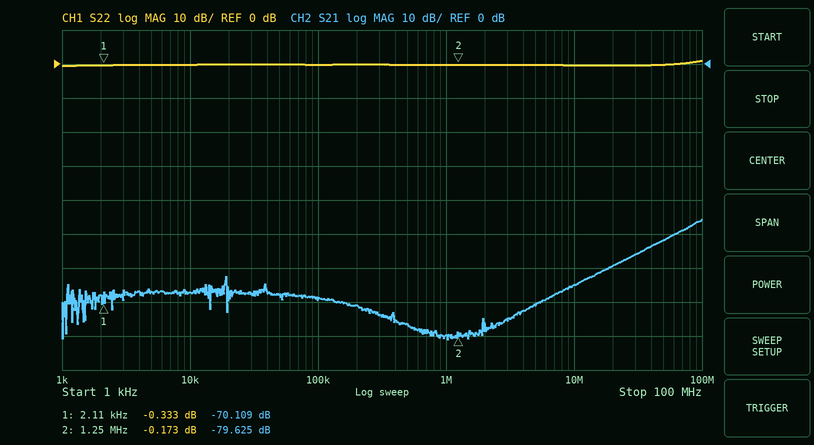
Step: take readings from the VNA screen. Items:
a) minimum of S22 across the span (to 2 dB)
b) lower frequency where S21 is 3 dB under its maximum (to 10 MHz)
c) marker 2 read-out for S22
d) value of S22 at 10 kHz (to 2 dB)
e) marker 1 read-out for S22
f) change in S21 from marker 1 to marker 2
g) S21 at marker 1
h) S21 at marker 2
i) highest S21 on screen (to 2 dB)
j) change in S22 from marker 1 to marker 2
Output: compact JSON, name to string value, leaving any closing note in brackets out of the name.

{"minimum of S22 across the span": "0 dB", "lower frequency where S21 is 3 dB under its maximum": "70 MHz", "marker 2 read-out for S22": "-0.173 dB", "value of S22 at 10 kHz": "0 dB", "marker 1 read-out for S22": "-0.333 dB", "change in S21 from marker 1 to marker 2": "-9.516 dB", "S21 at marker 1": "-70.109 dB", "S21 at marker 2": "-79.625 dB", "highest S21 on screen": "-46 dB", "change in S22 from marker 1 to marker 2": "0.160 dB"}
